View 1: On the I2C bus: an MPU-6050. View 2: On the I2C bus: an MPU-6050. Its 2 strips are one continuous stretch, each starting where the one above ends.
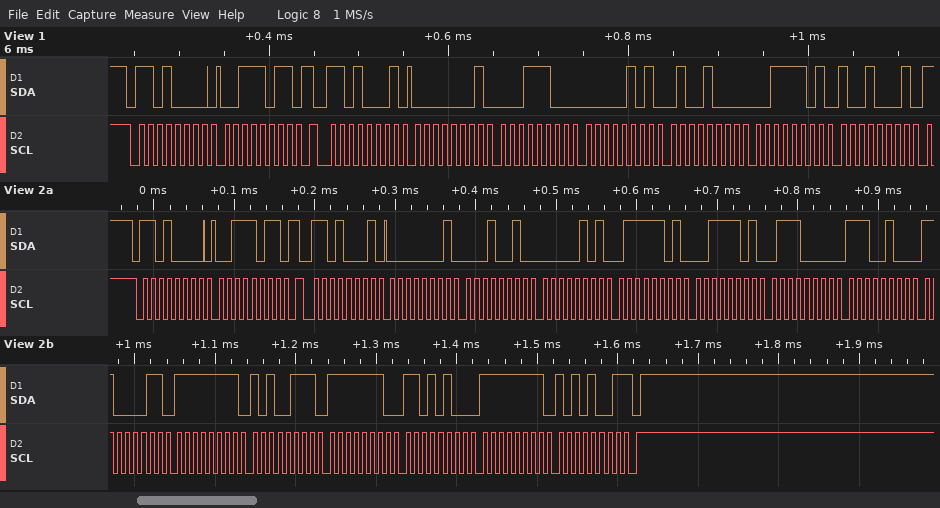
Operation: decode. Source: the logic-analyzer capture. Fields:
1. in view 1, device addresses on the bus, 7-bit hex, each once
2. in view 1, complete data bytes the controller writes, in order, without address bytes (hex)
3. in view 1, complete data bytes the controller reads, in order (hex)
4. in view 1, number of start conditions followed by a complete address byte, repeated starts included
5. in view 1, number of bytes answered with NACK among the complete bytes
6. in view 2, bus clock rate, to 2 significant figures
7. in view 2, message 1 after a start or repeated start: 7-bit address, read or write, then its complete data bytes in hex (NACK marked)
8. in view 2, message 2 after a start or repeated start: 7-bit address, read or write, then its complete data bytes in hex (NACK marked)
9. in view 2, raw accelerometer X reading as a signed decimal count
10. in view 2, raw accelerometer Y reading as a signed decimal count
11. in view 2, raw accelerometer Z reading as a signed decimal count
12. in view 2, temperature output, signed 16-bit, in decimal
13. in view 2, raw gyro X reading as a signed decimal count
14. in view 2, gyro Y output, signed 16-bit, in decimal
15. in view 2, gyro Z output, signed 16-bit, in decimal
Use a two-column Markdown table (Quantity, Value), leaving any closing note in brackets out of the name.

| Quantity | Value |
|---|---|
| in view 1, device addresses on the bus, 7-bit hex, each once | 0x68 |
| in view 1, complete data bytes the controller writes, in order, without address bytes | 3B |
| in view 1, complete data bytes the controller reads, in order | 01 1C 05 48 3D 91 |
| in view 1, number of start conditions followed by a complete address byte, repeated starts included | 2 |
| in view 1, number of bytes answered with NACK among the complete bytes | 0 |
| in view 2, bus clock rate, to 2 significant figures | 100 kHz |
| in view 2, message 1 after a start or repeated start: 7-bit address, read or write, then its complete data bytes in hex | 0x68 write: 3B |
| in view 2, message 2 after a start or repeated start: 7-bit address, read or write, then its complete data bytes in hex | 0x68 read: 01 12 05 7D 3D 70 E4 C3 FF A7 FE D4 FF A9 NACK |
| in view 2, raw accelerometer X reading as a signed decimal count | 274 |
| in view 2, raw accelerometer Y reading as a signed decimal count | 1405 |
| in view 2, raw accelerometer Z reading as a signed decimal count | 15728 |
| in view 2, temperature output, signed 16-bit, in decimal | -6973 |
| in view 2, raw gyro X reading as a signed decimal count | -89 |
| in view 2, gyro Y output, signed 16-bit, in decimal | -300 |
| in view 2, gyro Z output, signed 16-bit, in decimal | -87 |
